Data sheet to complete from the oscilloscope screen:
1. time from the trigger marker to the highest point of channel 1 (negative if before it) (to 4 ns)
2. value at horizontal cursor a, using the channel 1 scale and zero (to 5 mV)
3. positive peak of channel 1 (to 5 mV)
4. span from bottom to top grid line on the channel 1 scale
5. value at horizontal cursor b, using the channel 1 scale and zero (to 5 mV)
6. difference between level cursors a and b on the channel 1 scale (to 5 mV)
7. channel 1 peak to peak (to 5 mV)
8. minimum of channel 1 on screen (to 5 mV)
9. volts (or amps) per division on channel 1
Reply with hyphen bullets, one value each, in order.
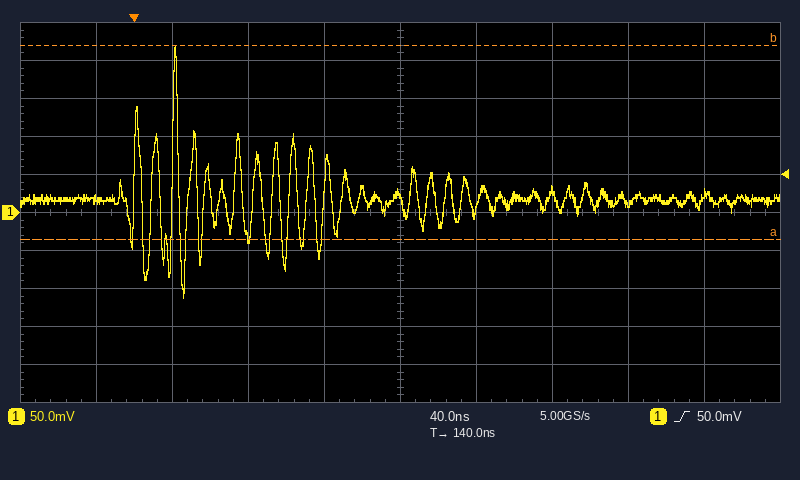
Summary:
- +20 ns
- -35 mV
- 220 mV
- 500 mV
- 220 mV
- 255 mV
- 330 mV
- -110 mV
- 50 mV
